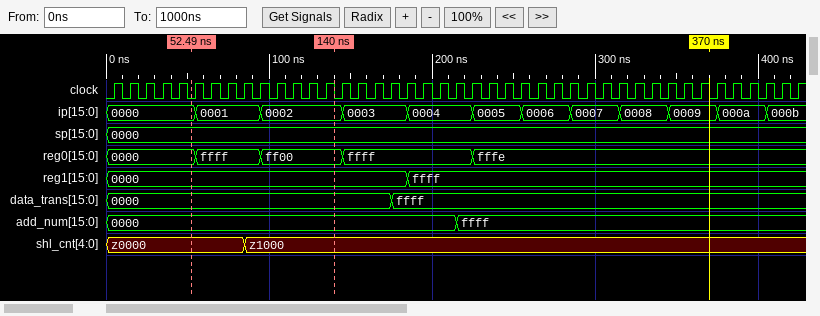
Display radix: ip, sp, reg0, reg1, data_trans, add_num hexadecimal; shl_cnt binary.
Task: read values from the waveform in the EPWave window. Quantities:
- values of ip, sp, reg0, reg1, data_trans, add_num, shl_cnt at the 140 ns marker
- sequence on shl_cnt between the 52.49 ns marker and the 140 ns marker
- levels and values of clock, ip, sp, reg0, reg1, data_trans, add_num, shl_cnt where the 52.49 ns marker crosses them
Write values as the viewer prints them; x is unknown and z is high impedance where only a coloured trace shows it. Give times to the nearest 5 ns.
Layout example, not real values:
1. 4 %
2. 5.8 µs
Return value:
1. ip=0002, sp=0000, reg0=ff00, reg1=0000, data_trans=0000, add_num=0000, shl_cnt=z1000
2. z0000, z1000
3. clock=0, ip=0000, sp=0000, reg0=0000, reg1=0000, data_trans=0000, add_num=0000, shl_cnt=z0000
